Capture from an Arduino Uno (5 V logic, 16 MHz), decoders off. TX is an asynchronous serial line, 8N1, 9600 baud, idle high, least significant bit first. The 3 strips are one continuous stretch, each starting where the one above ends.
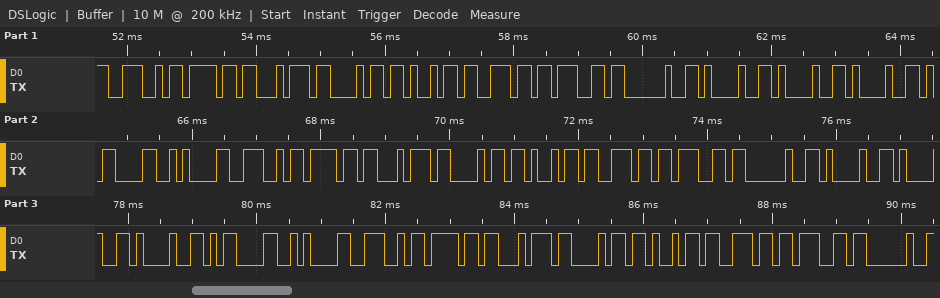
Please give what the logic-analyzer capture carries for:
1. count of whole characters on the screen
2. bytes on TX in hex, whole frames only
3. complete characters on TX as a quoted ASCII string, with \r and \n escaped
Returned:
34
4E 6F 74 68 69 6E 67 20 21 21 21 0D 0A 4E 6F 74 68 69 6E 67 20 21 21 21 0D 0A 4E 6F 74 68 69 6E 67 20
"Nothing !!!\r\nNothing !!!\r\nNothing "
